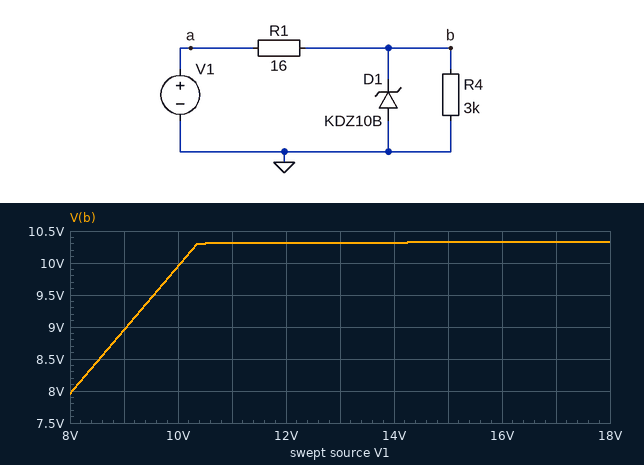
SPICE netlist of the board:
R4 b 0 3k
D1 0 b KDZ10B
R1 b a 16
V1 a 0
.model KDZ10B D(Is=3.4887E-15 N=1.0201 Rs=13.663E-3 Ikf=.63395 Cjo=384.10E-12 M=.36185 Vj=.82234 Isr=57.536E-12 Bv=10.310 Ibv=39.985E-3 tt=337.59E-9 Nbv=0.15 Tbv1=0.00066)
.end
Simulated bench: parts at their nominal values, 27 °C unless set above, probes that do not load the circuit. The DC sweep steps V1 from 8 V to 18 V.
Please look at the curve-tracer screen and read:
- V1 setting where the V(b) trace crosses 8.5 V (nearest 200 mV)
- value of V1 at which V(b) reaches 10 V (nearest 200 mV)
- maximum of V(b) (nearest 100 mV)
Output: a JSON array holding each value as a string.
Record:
["8.6 V", "10.0 V", "10.3 V"]
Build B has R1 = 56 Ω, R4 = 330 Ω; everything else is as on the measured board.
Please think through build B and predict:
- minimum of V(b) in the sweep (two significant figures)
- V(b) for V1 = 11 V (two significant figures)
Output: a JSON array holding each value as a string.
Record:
["6.8 V", "9.4 V"]
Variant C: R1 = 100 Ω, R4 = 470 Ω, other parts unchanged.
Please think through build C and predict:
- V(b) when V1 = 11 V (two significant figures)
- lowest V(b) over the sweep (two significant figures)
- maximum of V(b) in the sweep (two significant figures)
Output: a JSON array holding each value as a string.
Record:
["9.1 V", "6.6 V", "10 V"]
